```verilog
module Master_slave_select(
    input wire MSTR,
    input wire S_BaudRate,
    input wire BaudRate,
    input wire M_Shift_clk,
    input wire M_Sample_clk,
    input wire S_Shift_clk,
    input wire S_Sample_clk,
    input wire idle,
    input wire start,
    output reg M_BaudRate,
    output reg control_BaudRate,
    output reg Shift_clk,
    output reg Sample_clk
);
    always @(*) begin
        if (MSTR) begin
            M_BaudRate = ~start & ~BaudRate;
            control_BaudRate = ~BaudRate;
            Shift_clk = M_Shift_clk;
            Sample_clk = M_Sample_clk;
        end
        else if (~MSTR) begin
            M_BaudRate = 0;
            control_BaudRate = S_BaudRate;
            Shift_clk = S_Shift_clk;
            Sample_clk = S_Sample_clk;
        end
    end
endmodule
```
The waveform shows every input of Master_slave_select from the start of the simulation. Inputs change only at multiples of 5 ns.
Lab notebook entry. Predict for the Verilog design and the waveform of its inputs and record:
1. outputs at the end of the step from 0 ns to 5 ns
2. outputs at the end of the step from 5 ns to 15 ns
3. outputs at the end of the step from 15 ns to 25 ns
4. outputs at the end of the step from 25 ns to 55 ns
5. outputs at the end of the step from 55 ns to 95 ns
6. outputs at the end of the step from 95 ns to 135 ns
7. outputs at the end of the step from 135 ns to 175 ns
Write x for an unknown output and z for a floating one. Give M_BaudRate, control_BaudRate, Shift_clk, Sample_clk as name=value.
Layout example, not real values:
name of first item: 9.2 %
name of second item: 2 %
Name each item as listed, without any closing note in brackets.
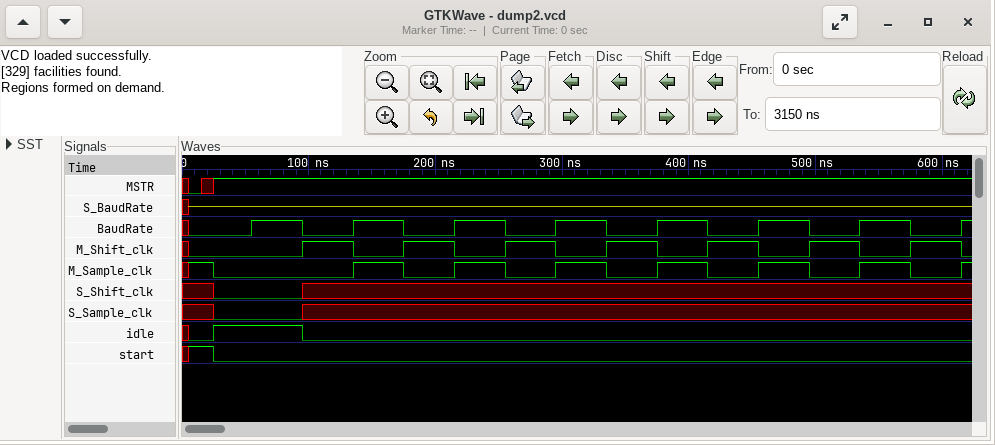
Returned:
outputs at the end of the step from 0 ns to 5 ns: M_BaudRate=x, control_BaudRate=x, Shift_clk=x, Sample_clk=x
outputs at the end of the step from 5 ns to 15 ns: M_BaudRate=0, control_BaudRate=z, Shift_clk=x, Sample_clk=x
outputs at the end of the step from 15 ns to 25 ns: M_BaudRate=0, control_BaudRate=z, Shift_clk=x, Sample_clk=x
outputs at the end of the step from 25 ns to 55 ns: M_BaudRate=1, control_BaudRate=1, Shift_clk=0, Sample_clk=0
outputs at the end of the step from 55 ns to 95 ns: M_BaudRate=0, control_BaudRate=0, Shift_clk=0, Sample_clk=0
outputs at the end of the step from 95 ns to 135 ns: M_BaudRate=1, control_BaudRate=1, Shift_clk=1, Sample_clk=0
outputs at the end of the step from 135 ns to 175 ns: M_BaudRate=0, control_BaudRate=0, Shift_clk=0, Sample_clk=1
